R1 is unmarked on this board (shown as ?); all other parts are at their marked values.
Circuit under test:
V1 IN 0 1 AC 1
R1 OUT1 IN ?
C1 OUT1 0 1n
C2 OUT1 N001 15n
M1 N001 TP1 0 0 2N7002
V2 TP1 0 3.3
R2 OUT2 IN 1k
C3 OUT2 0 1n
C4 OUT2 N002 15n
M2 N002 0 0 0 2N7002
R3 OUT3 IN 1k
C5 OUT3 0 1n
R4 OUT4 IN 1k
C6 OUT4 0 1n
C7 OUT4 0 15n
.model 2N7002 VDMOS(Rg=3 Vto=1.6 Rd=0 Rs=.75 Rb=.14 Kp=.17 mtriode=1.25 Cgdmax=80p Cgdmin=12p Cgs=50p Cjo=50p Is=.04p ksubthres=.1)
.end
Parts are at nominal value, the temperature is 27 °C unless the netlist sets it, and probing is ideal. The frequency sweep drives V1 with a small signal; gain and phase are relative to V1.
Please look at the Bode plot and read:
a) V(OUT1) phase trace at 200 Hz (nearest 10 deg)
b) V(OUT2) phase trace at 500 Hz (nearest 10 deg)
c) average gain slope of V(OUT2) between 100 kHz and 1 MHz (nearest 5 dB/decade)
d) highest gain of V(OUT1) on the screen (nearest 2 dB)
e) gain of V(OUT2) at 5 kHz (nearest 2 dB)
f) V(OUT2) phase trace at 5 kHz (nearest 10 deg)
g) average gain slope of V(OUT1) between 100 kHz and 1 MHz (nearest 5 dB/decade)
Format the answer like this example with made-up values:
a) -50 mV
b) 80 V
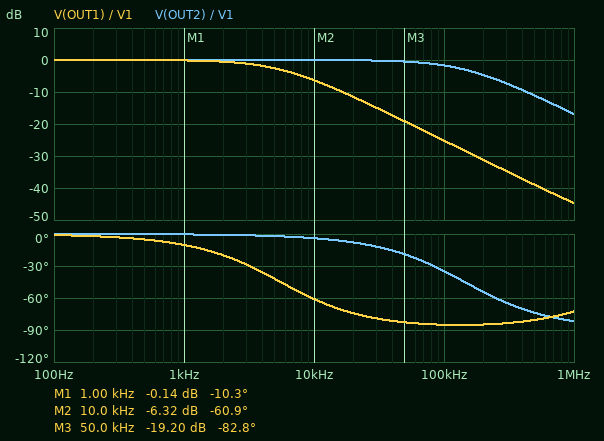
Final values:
a) 0 deg
b) 0 deg
c) -15 dB/decade
d) 0 dB
e) 0 dB
f) 0 deg
g) -20 dB/decade
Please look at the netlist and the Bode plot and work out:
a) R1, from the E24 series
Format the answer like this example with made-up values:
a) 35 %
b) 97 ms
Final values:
a) 1.8 kΩ
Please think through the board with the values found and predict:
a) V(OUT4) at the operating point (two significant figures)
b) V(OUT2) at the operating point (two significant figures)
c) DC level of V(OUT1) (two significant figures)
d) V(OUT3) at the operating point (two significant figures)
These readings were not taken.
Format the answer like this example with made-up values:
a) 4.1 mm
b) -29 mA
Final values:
a) 1.0 V
b) 1.0 V
c) 1.0 V
d) 1.0 V
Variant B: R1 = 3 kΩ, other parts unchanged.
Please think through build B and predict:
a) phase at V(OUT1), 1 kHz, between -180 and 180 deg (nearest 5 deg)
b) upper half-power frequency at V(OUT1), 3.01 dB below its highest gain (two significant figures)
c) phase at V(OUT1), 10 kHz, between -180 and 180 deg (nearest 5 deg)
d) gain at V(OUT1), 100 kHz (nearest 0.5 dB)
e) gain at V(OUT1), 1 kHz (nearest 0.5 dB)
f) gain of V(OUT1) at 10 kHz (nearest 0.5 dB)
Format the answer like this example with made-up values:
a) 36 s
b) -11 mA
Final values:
a) -15 deg
b) 3.3 kHz
c) -70 deg
d) -29.5 dB
e) -0.5 dB
f) -10.0 dB
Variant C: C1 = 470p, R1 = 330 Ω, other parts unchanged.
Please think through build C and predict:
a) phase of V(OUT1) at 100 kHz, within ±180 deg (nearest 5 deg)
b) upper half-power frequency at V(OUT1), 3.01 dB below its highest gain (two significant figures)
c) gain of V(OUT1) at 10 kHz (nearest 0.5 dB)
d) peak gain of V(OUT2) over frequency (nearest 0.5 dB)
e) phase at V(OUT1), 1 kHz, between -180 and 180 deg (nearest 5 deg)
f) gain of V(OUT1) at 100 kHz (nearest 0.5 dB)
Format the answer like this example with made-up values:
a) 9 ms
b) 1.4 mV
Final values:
a) -70 deg
b) 31 kHz
c) -0.5 dB
d) 0 dB
e) 0 deg
f) -10.5 dB
